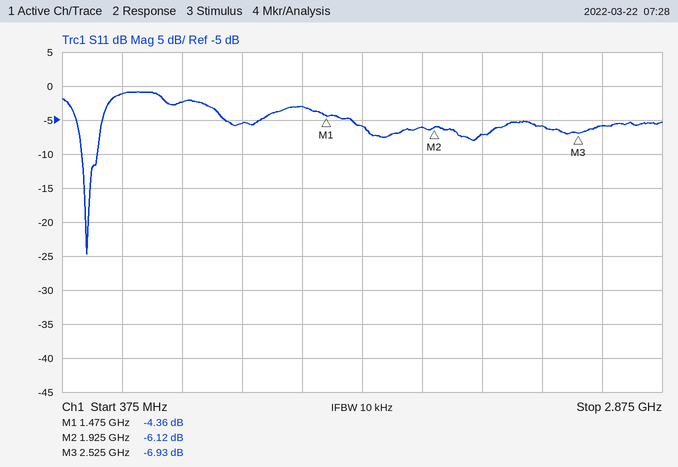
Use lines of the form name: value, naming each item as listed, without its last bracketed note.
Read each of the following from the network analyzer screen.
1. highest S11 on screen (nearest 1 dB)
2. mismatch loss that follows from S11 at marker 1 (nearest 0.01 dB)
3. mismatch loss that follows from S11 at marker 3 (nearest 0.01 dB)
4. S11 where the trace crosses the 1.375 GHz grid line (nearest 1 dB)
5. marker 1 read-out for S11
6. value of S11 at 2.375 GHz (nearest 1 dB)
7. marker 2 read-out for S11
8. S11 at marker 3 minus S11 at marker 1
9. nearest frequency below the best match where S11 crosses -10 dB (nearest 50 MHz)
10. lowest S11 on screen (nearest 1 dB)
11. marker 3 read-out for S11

highest S11 on screen: -1 dB
mismatch loss that follows from S11 at marker 1: 1.98 dB
mismatch loss that follows from S11 at marker 3: 0.98 dB
S11 where the trace crosses the 1.375 GHz grid line: -3 dB
marker 1 read-out for S11: -4.36 dB
value of S11 at 2.375 GHz: -6 dB
marker 2 read-out for S11: -6.12 dB
S11 at marker 3 minus S11 at marker 1: -2.57 dB
nearest frequency below the best match where S11 crosses -10 dB: 450 MHz
lowest S11 on screen: -25 dB
marker 3 read-out for S11: -6.93 dB
